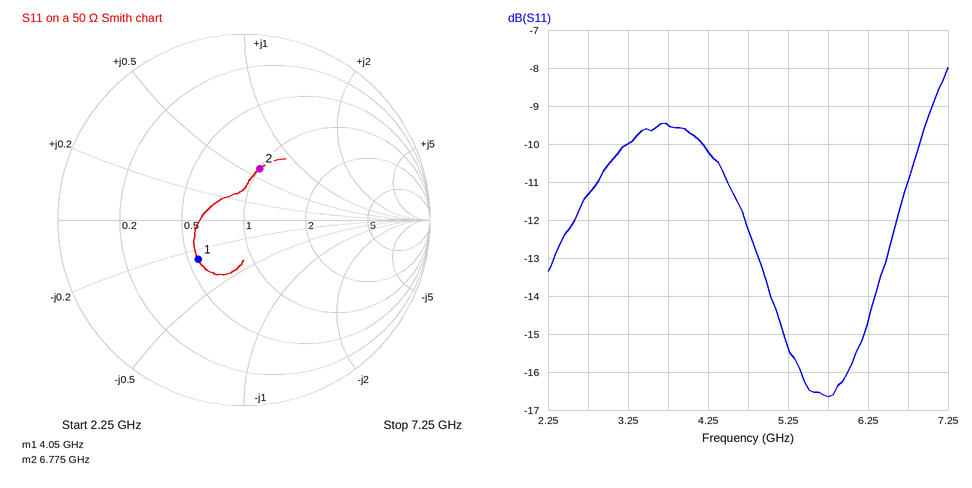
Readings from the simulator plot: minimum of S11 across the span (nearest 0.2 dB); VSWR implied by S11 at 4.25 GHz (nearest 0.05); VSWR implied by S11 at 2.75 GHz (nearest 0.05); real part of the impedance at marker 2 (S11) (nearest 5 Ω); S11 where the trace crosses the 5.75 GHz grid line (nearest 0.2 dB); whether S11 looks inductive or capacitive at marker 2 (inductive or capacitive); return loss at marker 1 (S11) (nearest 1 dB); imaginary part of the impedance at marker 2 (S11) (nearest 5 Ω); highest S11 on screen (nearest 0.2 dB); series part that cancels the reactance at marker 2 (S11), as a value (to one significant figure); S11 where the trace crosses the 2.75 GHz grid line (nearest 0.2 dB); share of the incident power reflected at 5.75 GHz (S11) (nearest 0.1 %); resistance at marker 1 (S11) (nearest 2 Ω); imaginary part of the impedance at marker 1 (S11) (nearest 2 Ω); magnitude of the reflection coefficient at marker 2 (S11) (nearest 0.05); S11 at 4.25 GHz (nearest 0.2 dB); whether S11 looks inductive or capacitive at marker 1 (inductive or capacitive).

-16.6 dB
1.90
1.75
50 Ω
-16.6 dB
inductive
10 dB
+30 Ω
-8.0 dB
800 fF
-11.4 dB
2.2 %
28 Ω
-14 Ω
0.30
-10.2 dB
capacitive
